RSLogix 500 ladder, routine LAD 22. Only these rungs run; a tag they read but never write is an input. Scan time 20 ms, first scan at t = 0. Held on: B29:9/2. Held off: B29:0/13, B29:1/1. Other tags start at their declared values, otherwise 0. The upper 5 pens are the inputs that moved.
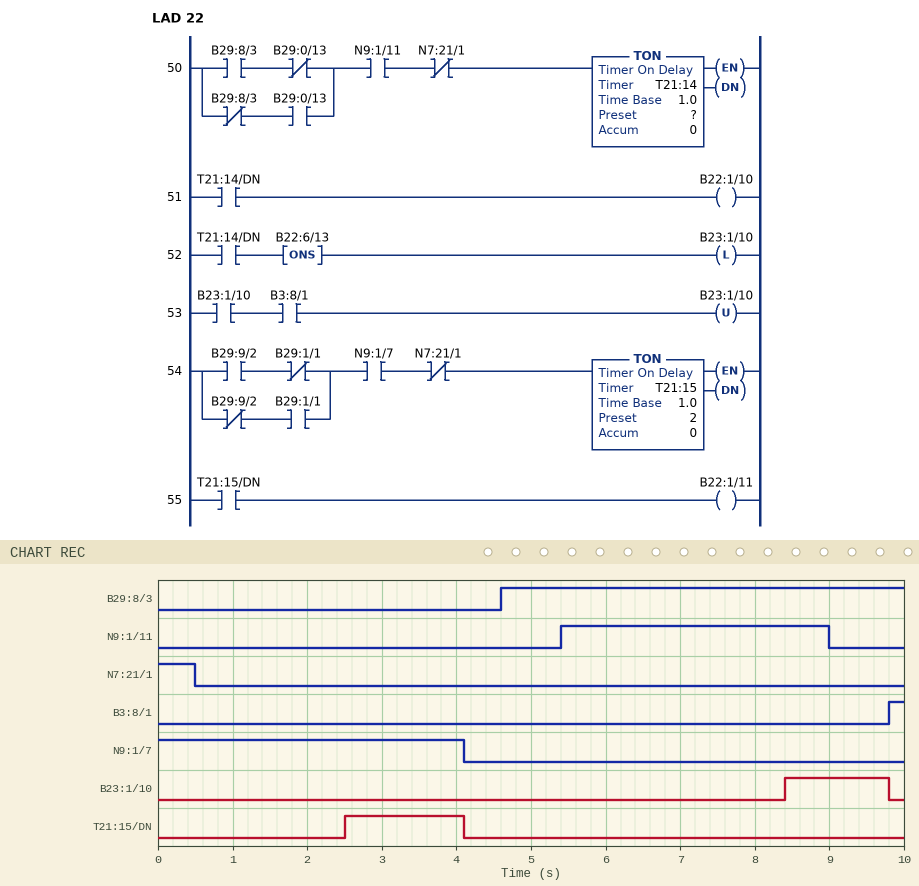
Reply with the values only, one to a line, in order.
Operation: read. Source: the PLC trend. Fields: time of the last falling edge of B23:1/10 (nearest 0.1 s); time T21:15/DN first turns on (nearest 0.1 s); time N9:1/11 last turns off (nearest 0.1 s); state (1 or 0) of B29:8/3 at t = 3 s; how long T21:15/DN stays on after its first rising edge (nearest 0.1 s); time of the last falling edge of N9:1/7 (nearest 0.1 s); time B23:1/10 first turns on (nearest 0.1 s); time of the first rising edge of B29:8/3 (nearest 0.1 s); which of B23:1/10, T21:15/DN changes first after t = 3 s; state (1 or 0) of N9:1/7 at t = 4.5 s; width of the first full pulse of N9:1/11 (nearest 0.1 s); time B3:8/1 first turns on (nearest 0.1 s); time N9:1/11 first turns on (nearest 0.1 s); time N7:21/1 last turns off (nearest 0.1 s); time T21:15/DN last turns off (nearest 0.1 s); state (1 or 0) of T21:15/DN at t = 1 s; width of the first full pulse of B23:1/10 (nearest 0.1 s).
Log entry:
9.8 s
2.5 s
9.0 s
0
1.6 s
4.1 s
8.4 s
4.6 s
T21:15/DN
0
3.6 s
9.8 s
5.4 s
0.5 s
4.1 s
0
1.4 s
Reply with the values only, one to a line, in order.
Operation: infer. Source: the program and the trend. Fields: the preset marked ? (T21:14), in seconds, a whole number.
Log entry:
3 s
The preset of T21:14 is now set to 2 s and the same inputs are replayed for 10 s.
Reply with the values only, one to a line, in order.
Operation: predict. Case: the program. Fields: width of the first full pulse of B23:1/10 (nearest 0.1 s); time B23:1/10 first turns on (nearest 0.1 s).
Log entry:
2.4 s
7.4 s
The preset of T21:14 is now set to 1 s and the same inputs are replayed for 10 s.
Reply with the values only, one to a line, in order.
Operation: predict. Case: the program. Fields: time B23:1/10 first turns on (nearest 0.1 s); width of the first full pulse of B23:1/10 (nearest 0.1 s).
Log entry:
6.4 s
3.4 s
